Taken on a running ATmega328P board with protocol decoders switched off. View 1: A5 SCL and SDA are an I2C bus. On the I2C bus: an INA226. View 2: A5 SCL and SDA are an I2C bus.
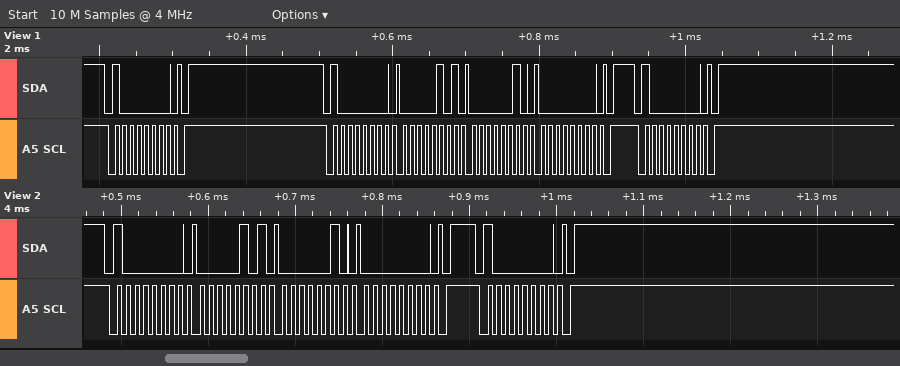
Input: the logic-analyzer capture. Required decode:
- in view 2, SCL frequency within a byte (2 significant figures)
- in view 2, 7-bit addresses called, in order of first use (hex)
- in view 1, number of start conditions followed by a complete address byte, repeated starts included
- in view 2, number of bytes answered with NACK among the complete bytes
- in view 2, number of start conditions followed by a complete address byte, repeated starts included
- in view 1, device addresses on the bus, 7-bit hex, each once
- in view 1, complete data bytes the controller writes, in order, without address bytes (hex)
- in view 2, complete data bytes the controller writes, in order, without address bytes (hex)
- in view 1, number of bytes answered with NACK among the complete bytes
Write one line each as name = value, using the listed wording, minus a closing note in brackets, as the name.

in view 2, SCL frequency within a byte = 100 kHz
in view 2, 7-bit addresses called, in order of first use = 0x40
in view 1, number of start conditions followed by a complete address byte, repeated starts included = 3
in view 2, number of bytes answered with NACK among the complete bytes = 0
in view 2, number of start conditions followed by a complete address byte, repeated starts included = 2
in view 1, device addresses on the bus, 7-bit hex, each once = 0x40
in view 1, complete data bytes the controller writes, in order, without address bytes = 05 02 00
in view 2, complete data bytes the controller writes, in order, without address bytes = 05 02 00
in view 1, number of bytes answered with NACK among the complete bytes = 0
